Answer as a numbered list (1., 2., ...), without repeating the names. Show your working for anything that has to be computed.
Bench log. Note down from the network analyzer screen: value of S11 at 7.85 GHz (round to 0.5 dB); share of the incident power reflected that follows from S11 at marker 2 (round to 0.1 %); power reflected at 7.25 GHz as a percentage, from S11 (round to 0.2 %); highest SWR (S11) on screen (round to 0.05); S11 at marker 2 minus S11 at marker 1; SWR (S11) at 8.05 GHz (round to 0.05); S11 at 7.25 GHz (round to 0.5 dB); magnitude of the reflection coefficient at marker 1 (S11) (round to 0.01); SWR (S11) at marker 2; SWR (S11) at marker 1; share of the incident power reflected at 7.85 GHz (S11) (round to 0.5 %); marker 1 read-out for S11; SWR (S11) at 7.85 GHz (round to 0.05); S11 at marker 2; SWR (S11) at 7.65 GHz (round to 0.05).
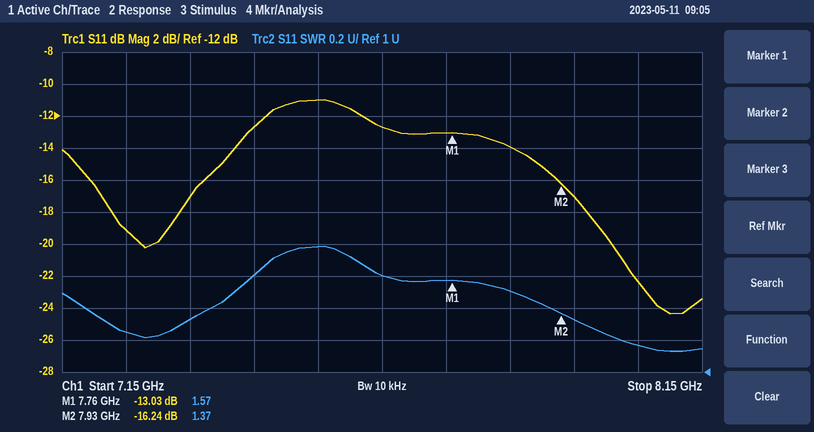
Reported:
1. -14.0 dB
2. 10^(-16.24/10) ≈ 2.4 %
3. 10^(-19/10) ≈ 1.26 %, so 1.2 % to the nearest 0.2 %
4. 1.80
5. -16.24 − (-13.03) = -3.21 dB
6. 1.15
7. -19.0 dB
8. 10^(-13.03/20) ≈ 0.22
9. 1.37
10. 1.57
11. 10^(-14/10) ≈ 4.0 %
12. -13.03 dB
13. 1.50
14. -16.24 dB
15. 1.60
